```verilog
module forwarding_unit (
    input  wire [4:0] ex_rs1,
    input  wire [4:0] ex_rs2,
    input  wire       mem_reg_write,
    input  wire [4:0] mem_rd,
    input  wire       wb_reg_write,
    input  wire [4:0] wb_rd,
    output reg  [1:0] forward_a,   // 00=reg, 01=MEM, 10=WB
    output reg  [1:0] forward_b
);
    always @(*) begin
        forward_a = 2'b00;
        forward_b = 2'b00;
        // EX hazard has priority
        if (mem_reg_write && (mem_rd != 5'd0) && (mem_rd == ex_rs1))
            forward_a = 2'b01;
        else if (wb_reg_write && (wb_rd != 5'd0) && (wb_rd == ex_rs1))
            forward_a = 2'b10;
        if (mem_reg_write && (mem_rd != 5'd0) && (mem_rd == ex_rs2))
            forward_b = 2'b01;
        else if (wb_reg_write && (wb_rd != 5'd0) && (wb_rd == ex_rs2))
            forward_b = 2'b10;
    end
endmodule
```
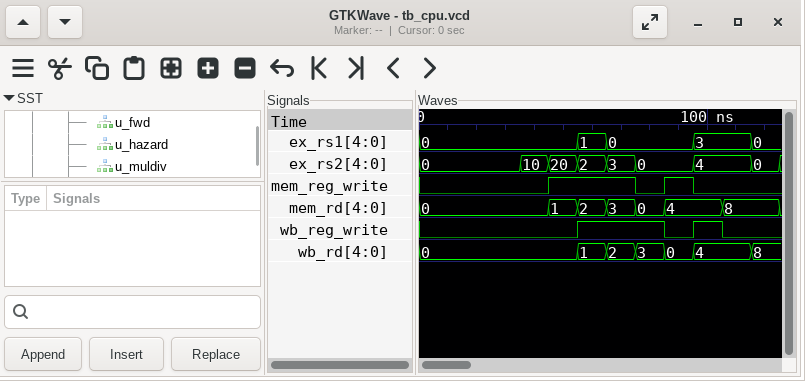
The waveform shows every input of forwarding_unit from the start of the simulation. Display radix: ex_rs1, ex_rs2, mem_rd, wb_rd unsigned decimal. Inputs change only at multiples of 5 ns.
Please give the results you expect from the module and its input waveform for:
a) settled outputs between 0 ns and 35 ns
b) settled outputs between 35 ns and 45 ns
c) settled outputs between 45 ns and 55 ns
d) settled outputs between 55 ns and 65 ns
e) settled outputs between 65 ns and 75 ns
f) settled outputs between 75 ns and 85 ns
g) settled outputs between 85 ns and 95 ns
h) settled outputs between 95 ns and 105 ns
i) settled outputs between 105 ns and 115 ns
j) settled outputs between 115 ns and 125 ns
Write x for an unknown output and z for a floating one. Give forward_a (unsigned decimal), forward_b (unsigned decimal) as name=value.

forward_a=0, forward_b=0
forward_a=0, forward_b=0
forward_a=0, forward_b=0
forward_a=2, forward_b=1
forward_a=0, forward_b=1
forward_a=0, forward_b=0
forward_a=0, forward_b=0
forward_a=0, forward_b=2
forward_a=0, forward_b=0
forward_a=0, forward_b=0
